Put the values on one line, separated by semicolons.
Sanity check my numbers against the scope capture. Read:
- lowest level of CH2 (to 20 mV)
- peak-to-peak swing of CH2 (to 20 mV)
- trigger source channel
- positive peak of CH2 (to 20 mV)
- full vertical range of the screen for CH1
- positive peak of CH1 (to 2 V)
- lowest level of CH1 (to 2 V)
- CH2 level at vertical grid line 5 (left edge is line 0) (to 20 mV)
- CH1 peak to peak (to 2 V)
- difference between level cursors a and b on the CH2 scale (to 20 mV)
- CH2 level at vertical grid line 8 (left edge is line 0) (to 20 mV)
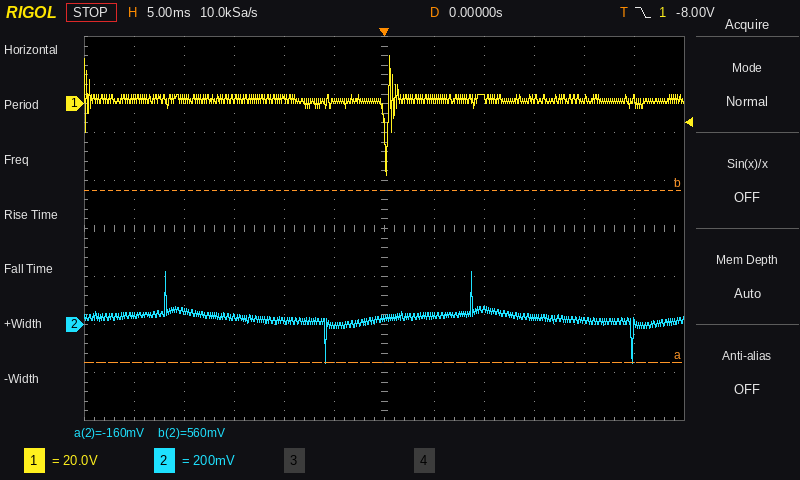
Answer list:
-160 mV; 380 mV; CH1; 220 mV; 160 V; 20 V; -30 V; 0 mV; 50 V; 720 mV; 60 mV
